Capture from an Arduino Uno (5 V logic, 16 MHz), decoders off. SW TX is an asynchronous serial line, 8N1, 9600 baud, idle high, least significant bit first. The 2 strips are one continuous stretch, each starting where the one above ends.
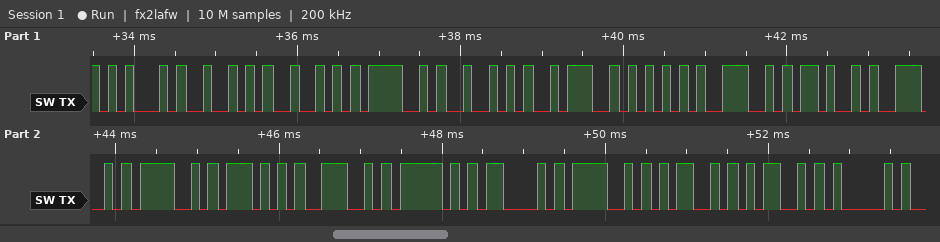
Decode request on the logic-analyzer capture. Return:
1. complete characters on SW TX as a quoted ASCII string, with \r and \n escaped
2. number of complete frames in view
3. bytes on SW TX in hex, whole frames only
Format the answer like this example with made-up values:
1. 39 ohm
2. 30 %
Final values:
1. "ERROR:UNKNOWN_COMMA"
2. 19
3. 45 52 52 4F 52 3A 55 4E 4B 4E 4F 57 4E 5F 43 4F 4D 4D 41
